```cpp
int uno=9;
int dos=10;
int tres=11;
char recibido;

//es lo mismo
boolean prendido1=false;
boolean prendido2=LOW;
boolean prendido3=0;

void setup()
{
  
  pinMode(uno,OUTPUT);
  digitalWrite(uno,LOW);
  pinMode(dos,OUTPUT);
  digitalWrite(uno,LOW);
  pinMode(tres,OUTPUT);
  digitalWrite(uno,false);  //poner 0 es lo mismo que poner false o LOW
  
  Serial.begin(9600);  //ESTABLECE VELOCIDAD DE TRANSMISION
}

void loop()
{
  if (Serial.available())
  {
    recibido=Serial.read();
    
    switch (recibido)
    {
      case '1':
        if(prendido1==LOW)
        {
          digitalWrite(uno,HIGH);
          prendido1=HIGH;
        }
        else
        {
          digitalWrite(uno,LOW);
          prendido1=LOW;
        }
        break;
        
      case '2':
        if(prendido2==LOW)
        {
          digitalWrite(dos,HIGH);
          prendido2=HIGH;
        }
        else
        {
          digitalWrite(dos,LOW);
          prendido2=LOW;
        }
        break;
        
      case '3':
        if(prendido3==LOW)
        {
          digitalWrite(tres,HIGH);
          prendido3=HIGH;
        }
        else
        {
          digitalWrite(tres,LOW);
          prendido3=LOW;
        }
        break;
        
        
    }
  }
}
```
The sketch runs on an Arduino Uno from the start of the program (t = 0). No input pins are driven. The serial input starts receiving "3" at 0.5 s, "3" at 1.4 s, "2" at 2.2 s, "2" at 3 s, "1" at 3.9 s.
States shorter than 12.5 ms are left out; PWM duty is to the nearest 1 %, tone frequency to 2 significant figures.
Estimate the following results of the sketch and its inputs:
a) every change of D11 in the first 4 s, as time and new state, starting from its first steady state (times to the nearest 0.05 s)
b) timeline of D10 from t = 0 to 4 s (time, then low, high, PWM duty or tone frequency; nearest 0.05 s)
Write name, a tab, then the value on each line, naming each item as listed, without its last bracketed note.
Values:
every change of D11 in the first 4 s, as time and new state, starting from its first steady state	0 s low; 0.5 s high; 1.4 s low
timeline of D10 from t = 0 to 4 s	0 s low; 2.2 s high; 3 s low
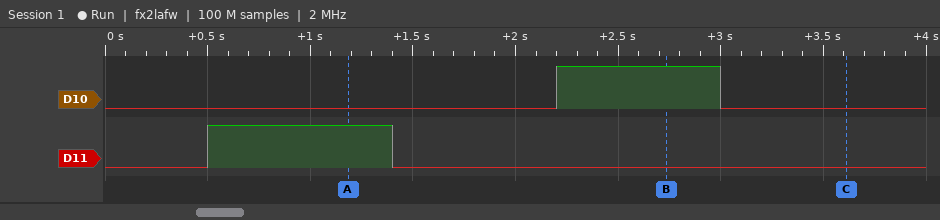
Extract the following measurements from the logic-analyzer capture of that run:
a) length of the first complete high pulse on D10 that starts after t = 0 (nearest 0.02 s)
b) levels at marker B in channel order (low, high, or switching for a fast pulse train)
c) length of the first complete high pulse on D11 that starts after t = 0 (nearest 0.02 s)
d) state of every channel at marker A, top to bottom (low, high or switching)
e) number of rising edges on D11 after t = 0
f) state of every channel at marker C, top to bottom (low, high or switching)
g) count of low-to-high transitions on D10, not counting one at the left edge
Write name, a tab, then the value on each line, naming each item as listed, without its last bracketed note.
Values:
length of the first complete high pulse on D10 that starts after t = 0	0.80 s
levels at marker B in channel order	D10 high, D11 low
length of the first complete high pulse on D11 that starts after t = 0	0.90 s
state of every channel at marker A, top to bottom	D10 low, D11 high
number of rising edges on D11 after t = 0	1
state of every channel at marker C, top to bottom	D10 low, D11 low
count of low-to-high transitions on D10, not counting one at the left edge	1
